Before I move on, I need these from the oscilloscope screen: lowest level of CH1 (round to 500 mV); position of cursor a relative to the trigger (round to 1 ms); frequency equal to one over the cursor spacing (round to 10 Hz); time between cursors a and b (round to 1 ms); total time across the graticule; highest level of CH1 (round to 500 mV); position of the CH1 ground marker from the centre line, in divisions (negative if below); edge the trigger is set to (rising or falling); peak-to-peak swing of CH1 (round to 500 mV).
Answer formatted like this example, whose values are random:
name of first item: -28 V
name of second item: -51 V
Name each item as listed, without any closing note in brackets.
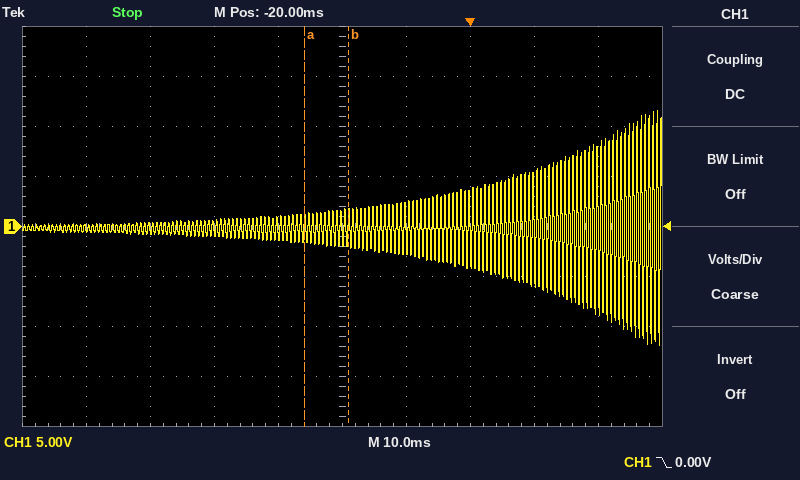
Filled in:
lowest level of CH1: -12.0 V
position of cursor a relative to the trigger: -26 ms
frequency equal to one over the cursor spacing: 140 Hz
time between cursors a and b: 7 ms
total time across the graticule: 100 ms
highest level of CH1: 11.5 V
position of the CH1 ground marker from the centre line, in divisions: 0.0 div
edge the trigger is set to: falling
peak-to-peak swing of CH1: 23.5 V
